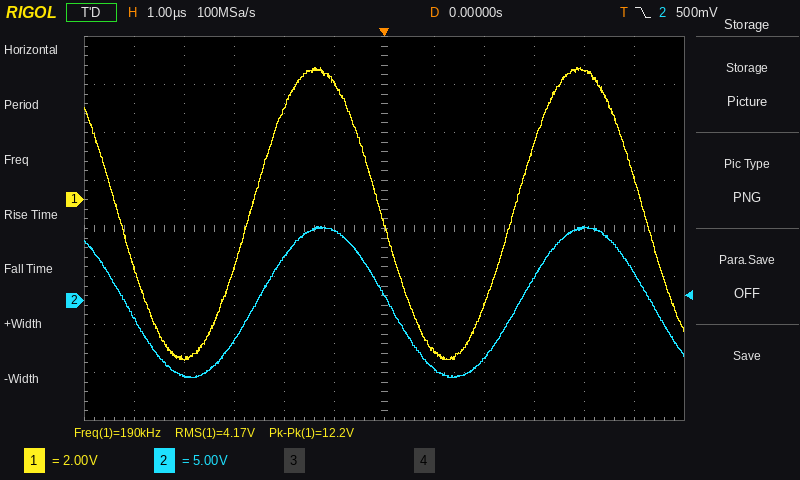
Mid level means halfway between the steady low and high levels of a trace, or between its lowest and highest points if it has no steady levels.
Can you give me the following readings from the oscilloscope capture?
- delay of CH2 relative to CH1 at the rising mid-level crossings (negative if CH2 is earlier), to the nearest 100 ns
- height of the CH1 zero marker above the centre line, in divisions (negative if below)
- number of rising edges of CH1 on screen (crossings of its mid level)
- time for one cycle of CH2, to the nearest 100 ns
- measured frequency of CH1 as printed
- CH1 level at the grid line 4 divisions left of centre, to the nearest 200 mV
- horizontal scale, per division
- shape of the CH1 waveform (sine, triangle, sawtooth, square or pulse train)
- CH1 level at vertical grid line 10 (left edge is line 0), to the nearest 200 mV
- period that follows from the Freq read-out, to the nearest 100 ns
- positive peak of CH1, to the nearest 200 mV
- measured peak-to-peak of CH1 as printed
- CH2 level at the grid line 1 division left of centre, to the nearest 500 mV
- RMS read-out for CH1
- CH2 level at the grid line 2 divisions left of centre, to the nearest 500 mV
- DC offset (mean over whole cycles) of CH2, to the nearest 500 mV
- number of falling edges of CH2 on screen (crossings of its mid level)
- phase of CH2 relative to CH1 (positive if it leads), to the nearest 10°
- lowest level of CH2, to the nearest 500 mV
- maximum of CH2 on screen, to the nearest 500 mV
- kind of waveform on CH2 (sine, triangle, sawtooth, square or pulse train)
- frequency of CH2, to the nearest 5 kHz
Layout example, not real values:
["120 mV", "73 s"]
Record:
["+100 ns", "+0.6 div", "2", "5.3 µs", "190 kHz", "-6.6 V", "1 µs", "sine", "5.4 V", "5.3 µs", "5.6 V", "12.2 V", "7.5 V", "4.17 V", "4.5 V", "0.0 V", "3", "-10°", "-8.0 V", "7.5 V", "sine", "190 kHz"]
